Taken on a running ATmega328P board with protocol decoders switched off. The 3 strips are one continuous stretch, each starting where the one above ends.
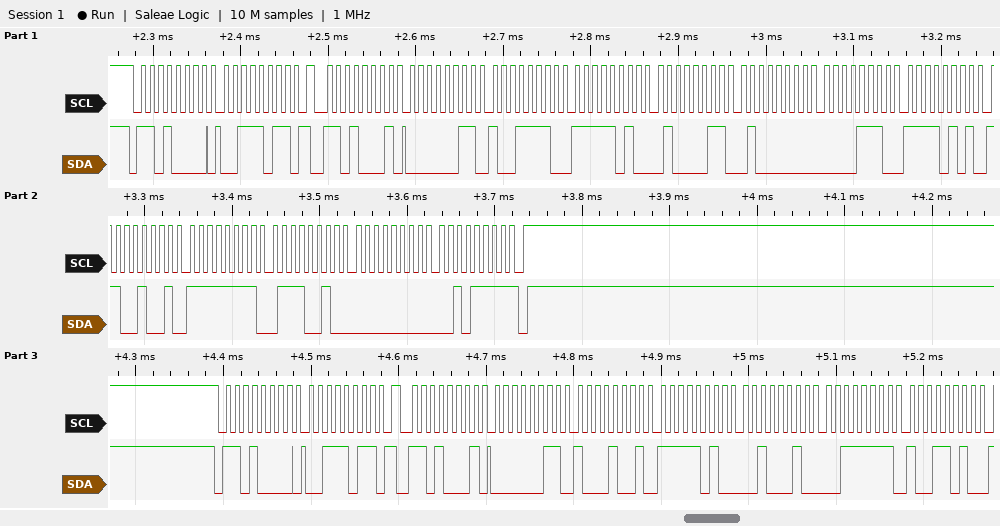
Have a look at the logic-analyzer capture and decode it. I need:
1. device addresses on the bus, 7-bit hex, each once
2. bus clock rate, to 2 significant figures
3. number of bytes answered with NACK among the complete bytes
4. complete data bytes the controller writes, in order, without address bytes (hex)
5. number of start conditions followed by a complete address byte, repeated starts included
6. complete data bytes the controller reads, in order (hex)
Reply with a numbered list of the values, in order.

1. 0x68
2. 100 kHz
3. 1
4. 3B 3B
5. 4
6. 03 9E FA 43 40 0E F5 C9 FF 72 00 2F 03 89 FA 22 3F 9A
